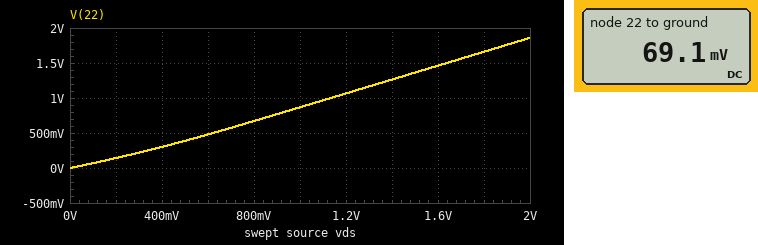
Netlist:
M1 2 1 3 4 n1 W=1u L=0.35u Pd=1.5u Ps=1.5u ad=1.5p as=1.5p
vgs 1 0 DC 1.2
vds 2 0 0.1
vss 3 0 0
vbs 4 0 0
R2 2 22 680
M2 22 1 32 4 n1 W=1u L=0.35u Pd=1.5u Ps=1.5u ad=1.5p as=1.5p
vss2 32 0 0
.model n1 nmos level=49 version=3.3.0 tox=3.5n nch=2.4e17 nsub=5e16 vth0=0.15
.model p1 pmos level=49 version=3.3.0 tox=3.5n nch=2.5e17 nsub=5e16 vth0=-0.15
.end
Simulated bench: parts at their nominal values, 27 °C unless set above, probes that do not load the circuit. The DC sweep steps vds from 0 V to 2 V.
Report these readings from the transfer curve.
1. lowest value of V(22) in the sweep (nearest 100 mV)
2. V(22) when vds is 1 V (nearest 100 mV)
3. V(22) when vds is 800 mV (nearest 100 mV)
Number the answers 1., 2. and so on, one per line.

1. 0 V
2. 900 mV
3. 700 mV
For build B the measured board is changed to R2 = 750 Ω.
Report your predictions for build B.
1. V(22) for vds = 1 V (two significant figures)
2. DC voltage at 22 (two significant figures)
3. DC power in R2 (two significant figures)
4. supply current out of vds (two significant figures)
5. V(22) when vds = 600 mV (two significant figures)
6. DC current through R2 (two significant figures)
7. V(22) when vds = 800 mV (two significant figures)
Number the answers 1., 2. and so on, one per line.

1. 850 mV
2. 67 mV
3. 1.5 µW
4. 110 µA
5. 470 mV
6. 44 µA
7. 660 mV
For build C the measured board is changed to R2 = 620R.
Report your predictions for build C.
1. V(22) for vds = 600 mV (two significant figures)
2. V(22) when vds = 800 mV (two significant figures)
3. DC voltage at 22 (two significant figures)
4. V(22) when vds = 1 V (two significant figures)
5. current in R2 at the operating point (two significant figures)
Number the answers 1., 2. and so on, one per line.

1. 490 mV
2. 680 mV
3. 71 mV
4. 880 mV
5. 47 µA
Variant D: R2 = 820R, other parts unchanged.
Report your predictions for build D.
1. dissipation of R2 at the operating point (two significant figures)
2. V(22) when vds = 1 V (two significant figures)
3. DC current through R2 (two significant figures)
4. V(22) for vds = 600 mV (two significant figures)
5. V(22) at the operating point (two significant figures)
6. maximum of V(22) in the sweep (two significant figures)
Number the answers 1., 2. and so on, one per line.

1. 1.5 µW
2. 840 mV
3. 43 µA
4. 460 mV
5. 65 mV
6. 1.8 V
